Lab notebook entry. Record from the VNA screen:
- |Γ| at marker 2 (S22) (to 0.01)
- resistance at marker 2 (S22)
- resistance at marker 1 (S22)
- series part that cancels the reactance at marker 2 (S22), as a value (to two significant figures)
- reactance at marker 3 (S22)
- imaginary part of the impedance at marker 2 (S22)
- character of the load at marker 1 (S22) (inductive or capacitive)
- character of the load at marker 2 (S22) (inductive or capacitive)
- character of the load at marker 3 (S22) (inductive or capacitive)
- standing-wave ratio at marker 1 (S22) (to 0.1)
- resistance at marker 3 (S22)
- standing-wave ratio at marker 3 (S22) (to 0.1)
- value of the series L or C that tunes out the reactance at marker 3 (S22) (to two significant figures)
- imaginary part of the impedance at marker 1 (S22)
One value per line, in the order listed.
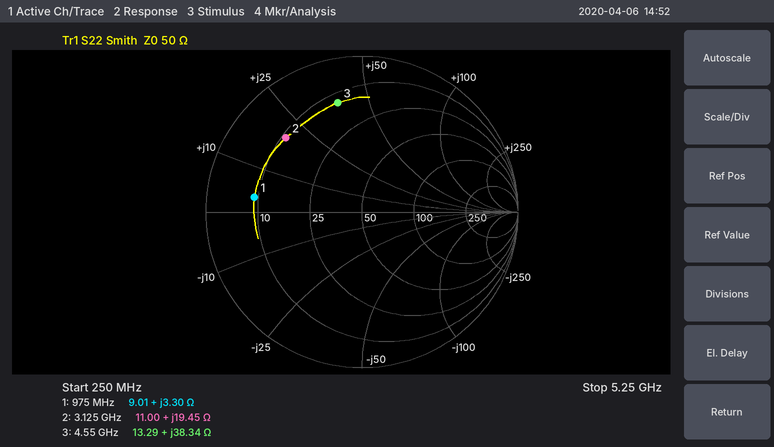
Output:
0.68
11.00 Ω
9.01 Ω
2.6 pF
+38.34 Ω
+19.45 Ω
inductive
inductive
inductive
5.6
13.29 Ω
6.1
910 fF
+3.30 Ω
